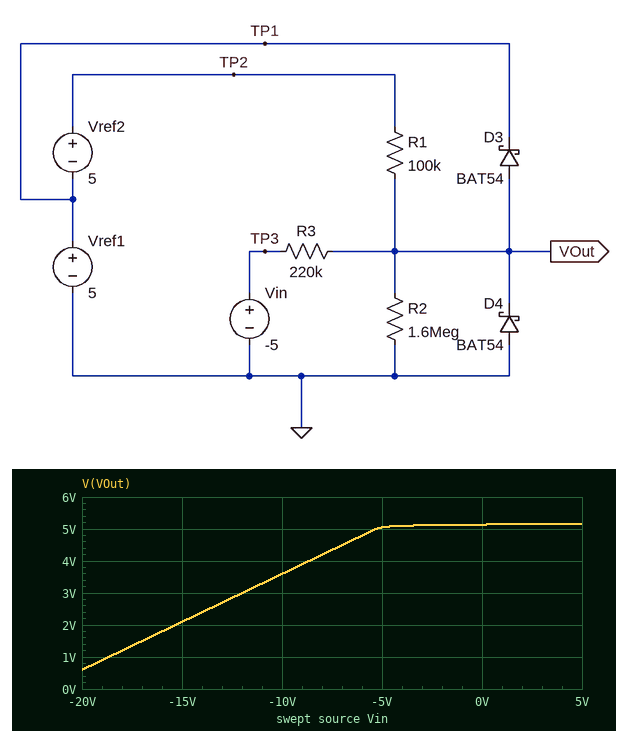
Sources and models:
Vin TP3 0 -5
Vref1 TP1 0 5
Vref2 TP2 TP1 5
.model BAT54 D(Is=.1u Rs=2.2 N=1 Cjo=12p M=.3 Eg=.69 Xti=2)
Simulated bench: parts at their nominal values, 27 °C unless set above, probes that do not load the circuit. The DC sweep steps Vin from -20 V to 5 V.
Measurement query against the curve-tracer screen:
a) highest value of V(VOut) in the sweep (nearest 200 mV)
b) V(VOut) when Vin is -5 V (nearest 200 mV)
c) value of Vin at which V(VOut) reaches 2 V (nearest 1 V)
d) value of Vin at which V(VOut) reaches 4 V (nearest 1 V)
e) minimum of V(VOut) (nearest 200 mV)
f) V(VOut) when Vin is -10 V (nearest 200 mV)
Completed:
5.2 V
5.0 V
-15 V
-9 V
600 mV
3.6 V
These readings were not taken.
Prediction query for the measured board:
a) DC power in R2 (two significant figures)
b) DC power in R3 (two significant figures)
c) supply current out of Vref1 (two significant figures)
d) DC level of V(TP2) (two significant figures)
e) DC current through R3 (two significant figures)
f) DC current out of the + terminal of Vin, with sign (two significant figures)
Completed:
16 µW
460 µW
49 µA
10 V
46 µA
-46 µA
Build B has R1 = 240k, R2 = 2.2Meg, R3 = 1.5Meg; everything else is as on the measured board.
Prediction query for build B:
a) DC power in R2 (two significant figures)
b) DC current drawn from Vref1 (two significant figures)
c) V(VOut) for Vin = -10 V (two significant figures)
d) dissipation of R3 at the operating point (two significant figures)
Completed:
12 µW
9.2 µA
5.1 V
68 µW
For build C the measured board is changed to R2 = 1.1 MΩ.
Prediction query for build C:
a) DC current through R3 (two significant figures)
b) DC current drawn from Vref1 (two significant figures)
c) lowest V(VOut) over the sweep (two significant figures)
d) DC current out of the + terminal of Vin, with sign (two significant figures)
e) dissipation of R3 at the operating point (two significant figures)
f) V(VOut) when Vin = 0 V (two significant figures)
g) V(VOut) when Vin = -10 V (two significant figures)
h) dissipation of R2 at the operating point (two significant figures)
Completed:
45 µA
50 µA
590 mV
-45 µA
450 µW
5.1 V
3.5 V
23 µW
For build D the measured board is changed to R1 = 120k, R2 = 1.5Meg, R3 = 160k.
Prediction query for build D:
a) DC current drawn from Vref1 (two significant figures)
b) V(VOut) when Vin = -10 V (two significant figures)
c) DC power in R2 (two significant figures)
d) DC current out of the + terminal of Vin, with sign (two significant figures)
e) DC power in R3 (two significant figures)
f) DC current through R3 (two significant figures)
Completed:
55 µA
1.4 V
7.8 µW
-53 µA
440 µW
53 µA
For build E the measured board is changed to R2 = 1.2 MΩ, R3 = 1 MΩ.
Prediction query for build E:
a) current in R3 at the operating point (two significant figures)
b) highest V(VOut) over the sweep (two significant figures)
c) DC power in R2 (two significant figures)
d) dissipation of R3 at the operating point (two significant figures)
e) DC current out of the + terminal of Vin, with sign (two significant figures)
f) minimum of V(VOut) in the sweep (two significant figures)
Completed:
10 µA
5.2 V
22 µW
100 µW
-10 µA
5.1 V
